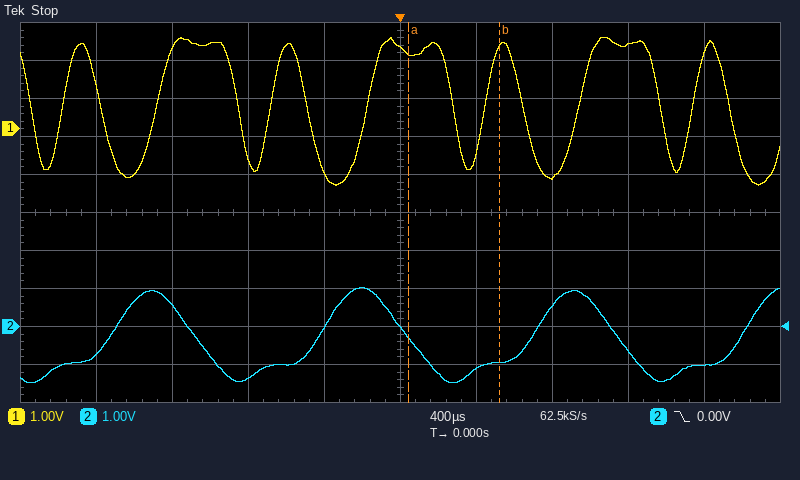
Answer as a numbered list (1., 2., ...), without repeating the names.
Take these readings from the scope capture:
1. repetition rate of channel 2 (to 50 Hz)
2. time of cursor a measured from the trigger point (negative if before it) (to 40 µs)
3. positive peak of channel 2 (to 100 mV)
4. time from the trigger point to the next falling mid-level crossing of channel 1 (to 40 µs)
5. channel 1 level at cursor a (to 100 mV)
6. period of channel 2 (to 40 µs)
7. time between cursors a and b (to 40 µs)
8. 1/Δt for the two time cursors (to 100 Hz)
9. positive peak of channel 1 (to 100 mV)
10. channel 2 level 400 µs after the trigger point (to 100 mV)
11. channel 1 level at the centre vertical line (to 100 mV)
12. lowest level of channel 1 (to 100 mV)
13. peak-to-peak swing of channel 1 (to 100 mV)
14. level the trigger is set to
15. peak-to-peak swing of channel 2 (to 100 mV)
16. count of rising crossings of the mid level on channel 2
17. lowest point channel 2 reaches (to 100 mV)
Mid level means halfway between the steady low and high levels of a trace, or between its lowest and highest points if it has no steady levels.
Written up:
1. 900 Hz
2. +40 µs
3. 1.0 V
4. 280 µs
5. 2.0 V
6. 1.12 ms
7. 480 µs
8. 2.1 kHz
9. 2.4 V
10. -1.1 V
11. 2.1 V
12. -1.5 V
13. 3.9 V
14. 0.00 V
15. 2.5 V
16. 4
17. -1.5 V
